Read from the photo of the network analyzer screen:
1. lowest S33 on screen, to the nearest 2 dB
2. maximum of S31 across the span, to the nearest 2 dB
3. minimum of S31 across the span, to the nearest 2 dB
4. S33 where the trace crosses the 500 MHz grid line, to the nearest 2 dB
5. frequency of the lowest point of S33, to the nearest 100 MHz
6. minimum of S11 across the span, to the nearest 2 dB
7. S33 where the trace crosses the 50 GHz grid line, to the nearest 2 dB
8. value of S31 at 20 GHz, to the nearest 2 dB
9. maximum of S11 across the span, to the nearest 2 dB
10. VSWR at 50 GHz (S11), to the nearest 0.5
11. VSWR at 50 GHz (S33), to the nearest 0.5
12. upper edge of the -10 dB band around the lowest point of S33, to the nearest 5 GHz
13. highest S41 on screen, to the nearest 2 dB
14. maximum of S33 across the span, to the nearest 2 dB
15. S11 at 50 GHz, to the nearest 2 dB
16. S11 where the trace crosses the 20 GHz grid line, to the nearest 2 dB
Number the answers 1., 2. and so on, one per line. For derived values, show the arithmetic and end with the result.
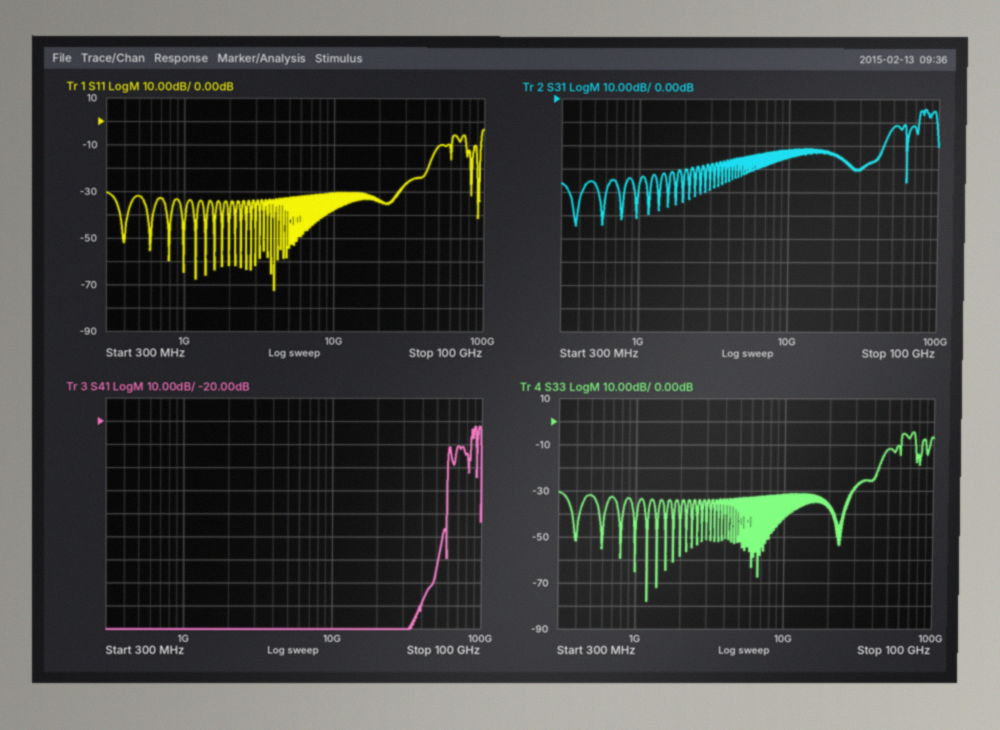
1. -78 dB
2. -4 dB
3. -54 dB
4. -32 dB
5. 1.2 GHz
6. -72 dB
7. -12 dB
8. -24 dB
9. -4 dB
10. |Γ| = 10^(-10/20) = 0.3162; VSWR = (1 + 0.3162)/(1 − 0.3162) ≈ 1.92, so 2.0 to the nearest 0.5
11. |Γ| = 10^(-12/20) = 0.2512; VSWR = (1 + 0.2512)/(1 − 0.2512) ≈ 1.67, so 1.5 to the nearest 0.5
12. 60 GHz
13. -22 dB
14. -4 dB
15. -10 dB
16. -34 dB
